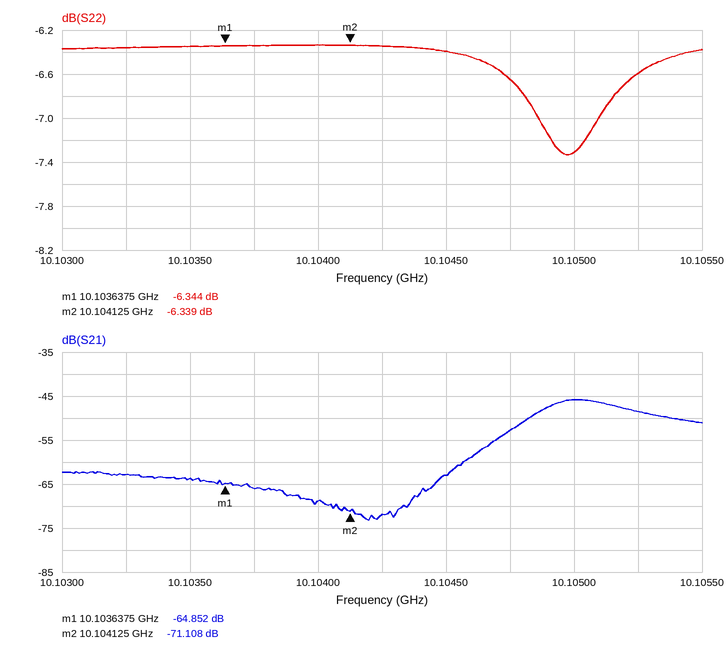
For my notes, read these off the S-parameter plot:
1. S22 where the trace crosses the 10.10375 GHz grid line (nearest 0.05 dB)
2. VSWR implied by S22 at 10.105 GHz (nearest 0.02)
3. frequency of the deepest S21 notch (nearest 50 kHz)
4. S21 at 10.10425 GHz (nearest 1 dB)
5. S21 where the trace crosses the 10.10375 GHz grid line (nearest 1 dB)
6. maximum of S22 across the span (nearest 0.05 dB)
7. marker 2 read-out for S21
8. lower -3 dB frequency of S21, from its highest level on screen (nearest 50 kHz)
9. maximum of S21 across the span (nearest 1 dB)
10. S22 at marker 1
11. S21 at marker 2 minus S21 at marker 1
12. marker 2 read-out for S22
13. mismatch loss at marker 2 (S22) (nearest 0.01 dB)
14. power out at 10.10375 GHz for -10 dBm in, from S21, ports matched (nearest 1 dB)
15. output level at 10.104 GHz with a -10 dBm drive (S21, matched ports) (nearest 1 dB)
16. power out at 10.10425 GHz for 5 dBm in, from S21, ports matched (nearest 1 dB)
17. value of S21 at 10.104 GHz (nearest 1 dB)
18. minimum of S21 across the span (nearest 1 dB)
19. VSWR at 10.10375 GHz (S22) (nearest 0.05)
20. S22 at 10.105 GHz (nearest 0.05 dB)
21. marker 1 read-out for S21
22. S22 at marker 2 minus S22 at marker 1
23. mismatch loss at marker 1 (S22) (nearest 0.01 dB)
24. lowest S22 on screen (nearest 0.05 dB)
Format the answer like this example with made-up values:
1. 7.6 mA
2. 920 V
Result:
1. -6.35 dB
2. 2.52
3. 10.10420 GHz
4. -72 dB
5. -66 dB
6. -6.35 dB
7. -71.108 dB
8. 10.10485 GHz
9. -46 dB
10. -6.344 dB
11. -6.256 dB
12. -6.339 dB
13. 1.15 dB
14. -76 dBm
15. -79 dBm
16. -67 dBm
17. -69 dB
18. -73 dB
19. 2.85
20. -7.30 dB
21. -64.852 dB
22. 0.005 dB
23. 1.15 dB
24. -7.35 dB
